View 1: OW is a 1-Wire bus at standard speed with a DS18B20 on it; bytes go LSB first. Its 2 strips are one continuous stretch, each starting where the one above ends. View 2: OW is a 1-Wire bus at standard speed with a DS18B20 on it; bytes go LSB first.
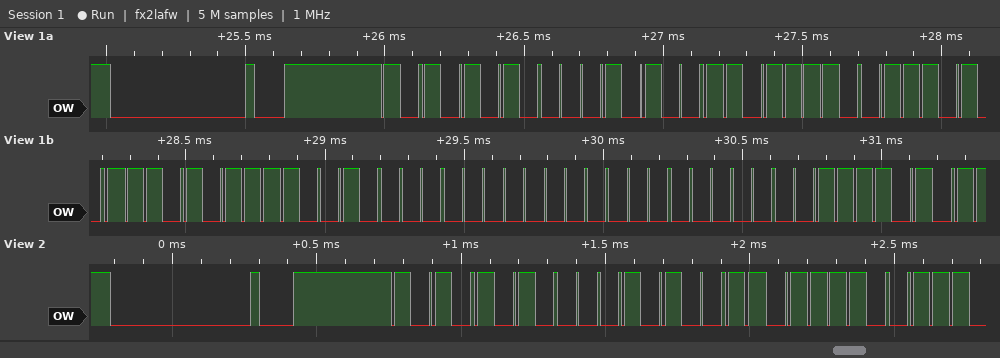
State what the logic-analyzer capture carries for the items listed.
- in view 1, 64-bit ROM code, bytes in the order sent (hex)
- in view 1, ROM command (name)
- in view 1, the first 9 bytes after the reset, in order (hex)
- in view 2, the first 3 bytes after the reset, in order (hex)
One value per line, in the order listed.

28 7B AE EB 09 00 00 BC
Match ROM
55 28 7B AE EB 09 00 00 BC
55 28 7B
